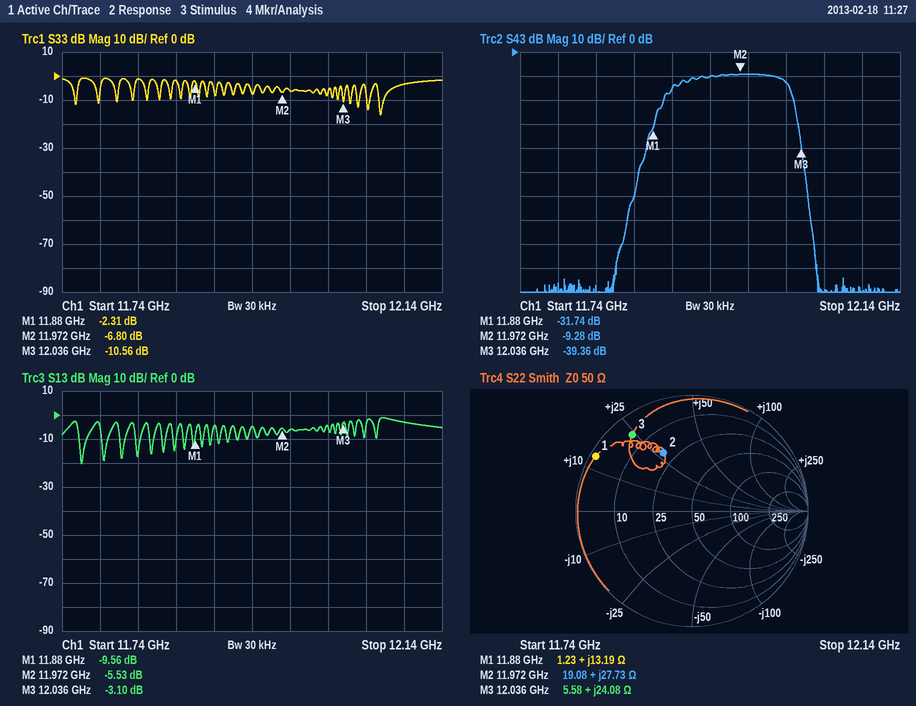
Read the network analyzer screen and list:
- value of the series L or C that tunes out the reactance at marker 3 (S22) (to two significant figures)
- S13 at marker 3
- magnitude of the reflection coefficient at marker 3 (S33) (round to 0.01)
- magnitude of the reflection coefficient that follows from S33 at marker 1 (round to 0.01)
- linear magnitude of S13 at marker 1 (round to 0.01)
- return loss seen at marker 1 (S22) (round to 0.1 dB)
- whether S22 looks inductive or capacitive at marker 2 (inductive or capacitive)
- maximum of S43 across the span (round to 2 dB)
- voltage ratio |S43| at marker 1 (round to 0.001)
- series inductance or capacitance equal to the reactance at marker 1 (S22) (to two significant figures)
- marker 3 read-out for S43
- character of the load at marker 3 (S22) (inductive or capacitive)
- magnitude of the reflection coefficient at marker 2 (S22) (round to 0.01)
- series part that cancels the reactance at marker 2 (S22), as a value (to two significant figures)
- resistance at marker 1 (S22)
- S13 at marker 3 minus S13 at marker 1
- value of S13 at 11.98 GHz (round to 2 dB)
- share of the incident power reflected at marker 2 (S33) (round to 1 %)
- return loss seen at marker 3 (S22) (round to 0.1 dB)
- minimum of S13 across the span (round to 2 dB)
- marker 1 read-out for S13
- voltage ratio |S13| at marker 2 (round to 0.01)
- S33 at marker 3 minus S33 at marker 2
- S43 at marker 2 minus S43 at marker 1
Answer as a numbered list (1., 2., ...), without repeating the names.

1. 550 fF
2. -3.10 dB
3. 0.30
4. 0.77
5. 0.33
6. 0.4 dB
7. inductive
8. -10 dB
9. 0.026
10. 180 pH
11. -39.36 dB
12. inductive
13. 0.56
14. 480 fF
15. 1.23 Ω
16. 6.46 dB
17. -6 dB
18. 21 %
19. 1.6 dB
20. -20 dB
21. -9.56 dB
22. 0.53
23. -3.76 dB
24. 22.46 dB
